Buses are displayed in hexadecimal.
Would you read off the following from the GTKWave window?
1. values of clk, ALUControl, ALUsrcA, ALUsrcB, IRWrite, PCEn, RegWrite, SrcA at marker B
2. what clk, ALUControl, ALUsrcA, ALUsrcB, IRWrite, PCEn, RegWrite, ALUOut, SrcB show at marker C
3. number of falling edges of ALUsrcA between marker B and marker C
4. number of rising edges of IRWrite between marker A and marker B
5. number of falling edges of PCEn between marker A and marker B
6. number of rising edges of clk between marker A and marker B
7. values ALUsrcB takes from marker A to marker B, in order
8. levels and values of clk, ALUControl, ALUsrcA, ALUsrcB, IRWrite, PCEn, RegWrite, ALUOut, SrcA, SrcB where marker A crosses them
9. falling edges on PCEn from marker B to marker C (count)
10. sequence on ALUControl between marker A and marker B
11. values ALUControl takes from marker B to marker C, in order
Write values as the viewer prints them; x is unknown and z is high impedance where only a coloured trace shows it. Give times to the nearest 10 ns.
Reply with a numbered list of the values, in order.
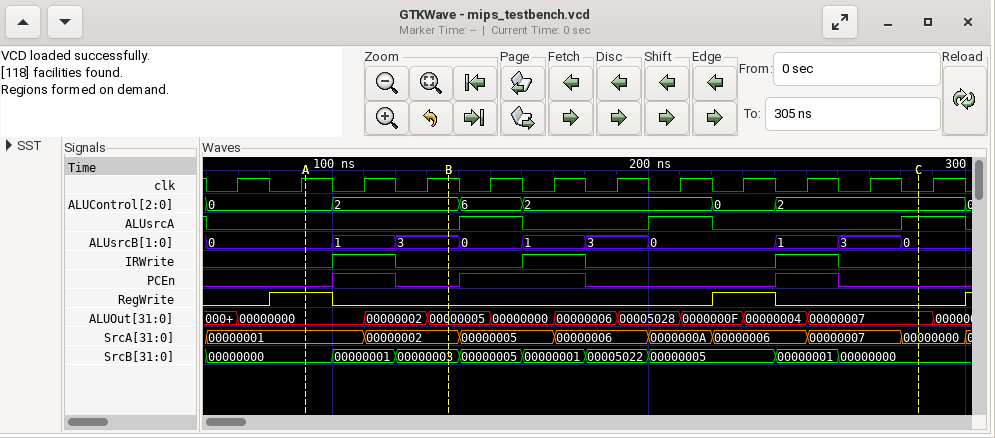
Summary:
1. clk=1, ALUControl=2, ALUsrcA=0, ALUsrcB=3, IRWrite=0, PCEn=0, RegWrite=0, SrcA=00000002
2. clk=0, ALUControl=2, ALUsrcA=1, ALUsrcB=0, IRWrite=0, PCEn=0, RegWrite=0, ALUOut=00000007, SrcB=00000000
3. 2
4. 1
5. 1
6. 2
7. 0, 1, 3
8. clk=1, ALUControl=0, ALUsrcA=0, ALUsrcB=0, IRWrite=0, PCEn=0, RegWrite=1, ALUOut=00000000, SrcA=00000001, SrcB=00000000
9. 2
10. 0, 2
11. 2, 6, 2, 0, 2
